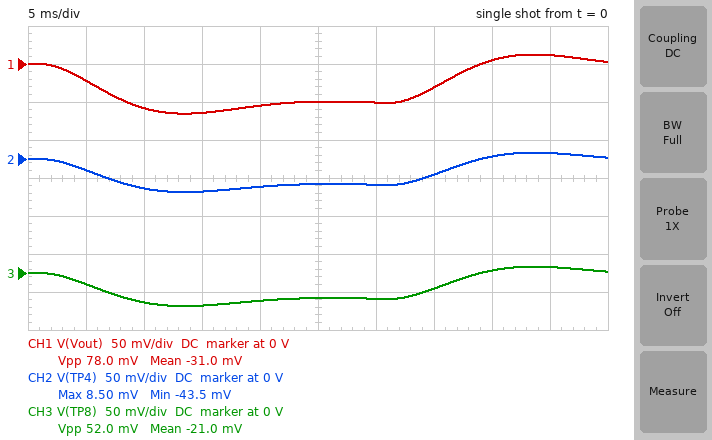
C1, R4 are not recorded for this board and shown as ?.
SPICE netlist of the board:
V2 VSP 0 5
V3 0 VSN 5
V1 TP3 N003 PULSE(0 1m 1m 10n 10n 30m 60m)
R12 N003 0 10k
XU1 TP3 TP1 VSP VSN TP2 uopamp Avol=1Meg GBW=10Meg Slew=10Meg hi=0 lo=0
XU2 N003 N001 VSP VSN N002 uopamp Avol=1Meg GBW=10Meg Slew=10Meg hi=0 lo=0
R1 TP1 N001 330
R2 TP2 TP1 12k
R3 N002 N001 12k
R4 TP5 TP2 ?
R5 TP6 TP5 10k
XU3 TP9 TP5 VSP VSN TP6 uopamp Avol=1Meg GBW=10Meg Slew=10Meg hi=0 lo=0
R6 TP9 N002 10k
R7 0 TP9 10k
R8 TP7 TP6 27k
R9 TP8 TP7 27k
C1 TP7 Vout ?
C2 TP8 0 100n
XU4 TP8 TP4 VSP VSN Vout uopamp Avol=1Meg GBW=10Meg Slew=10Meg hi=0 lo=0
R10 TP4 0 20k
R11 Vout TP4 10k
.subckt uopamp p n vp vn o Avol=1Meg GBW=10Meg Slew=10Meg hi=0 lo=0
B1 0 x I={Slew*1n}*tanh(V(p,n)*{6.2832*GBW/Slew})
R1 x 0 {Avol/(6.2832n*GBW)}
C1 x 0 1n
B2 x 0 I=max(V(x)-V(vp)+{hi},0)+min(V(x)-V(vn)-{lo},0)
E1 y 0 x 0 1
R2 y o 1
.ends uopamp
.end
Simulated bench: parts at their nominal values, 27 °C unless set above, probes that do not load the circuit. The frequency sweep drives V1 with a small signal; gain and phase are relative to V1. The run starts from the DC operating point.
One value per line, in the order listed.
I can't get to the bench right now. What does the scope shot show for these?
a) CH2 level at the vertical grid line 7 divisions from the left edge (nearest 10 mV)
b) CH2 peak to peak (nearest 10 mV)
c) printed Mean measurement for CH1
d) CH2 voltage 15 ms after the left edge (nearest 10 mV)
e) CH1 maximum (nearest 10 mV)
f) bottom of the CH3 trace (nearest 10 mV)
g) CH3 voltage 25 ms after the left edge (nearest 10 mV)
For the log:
-20 mV
50 mV
-31.0 mV
-40 mV
10 mV
-40 mV
-30 mV
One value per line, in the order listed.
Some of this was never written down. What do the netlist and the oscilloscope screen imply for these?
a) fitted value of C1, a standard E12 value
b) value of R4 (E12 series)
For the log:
180 nF
33 kΩ
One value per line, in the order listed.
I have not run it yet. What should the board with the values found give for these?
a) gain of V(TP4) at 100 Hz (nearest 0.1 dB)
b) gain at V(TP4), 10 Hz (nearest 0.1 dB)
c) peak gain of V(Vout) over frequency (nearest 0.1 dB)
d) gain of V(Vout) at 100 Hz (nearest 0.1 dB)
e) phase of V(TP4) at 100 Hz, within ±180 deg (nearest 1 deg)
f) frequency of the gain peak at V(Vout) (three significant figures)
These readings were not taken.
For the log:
17.7 dB
31.2 dB
36.9 dB
21.2 dB
24 deg
35.8 Hz
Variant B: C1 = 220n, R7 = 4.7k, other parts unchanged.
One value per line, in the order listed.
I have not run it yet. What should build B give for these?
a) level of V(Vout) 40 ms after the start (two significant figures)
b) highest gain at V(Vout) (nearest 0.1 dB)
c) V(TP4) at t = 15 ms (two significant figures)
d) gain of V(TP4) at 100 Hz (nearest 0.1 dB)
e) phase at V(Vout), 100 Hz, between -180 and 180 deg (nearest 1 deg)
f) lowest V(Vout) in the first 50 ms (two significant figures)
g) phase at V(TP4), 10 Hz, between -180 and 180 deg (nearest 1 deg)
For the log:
3.5 mV
36.7 dB
-36 mV
13.6 dB
16 deg
-54 mV
171 deg
